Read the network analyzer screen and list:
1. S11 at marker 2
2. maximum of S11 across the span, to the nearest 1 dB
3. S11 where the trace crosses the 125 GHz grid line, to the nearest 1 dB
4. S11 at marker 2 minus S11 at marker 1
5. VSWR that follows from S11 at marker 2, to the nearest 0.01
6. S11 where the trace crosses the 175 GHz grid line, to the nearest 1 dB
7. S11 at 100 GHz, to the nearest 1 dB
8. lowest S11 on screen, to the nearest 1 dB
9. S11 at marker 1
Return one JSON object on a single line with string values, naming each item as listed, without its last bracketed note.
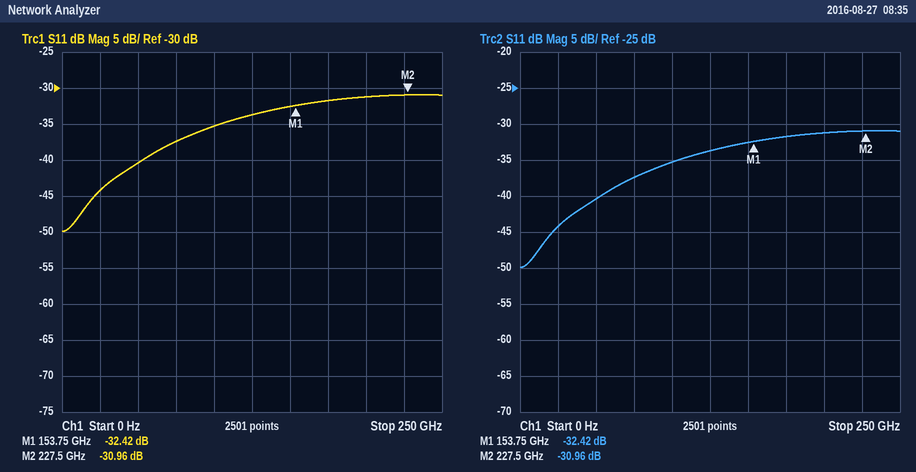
{"S11 at marker 2": "-30.96 dB", "maximum of S11 across the span, to the nearest 1 dB": "-31 dB", "S11 where the trace crosses the 125 GHz grid line, to the nearest 1 dB": "-34 dB", "S11 at marker 2 minus S11 at marker 1": "1.46 dB", "VSWR that follows from S11 at marker 2, to the nearest 0.01": "1.06", "S11 where the trace crosses the 175 GHz grid line, to the nearest 1 dB": "-32 dB", "S11 at 100 GHz, to the nearest 1 dB": "-35 dB", "lowest S11 on screen, to the nearest 1 dB": "-50 dB", "S11 at marker 1": "-32.42 dB"}
